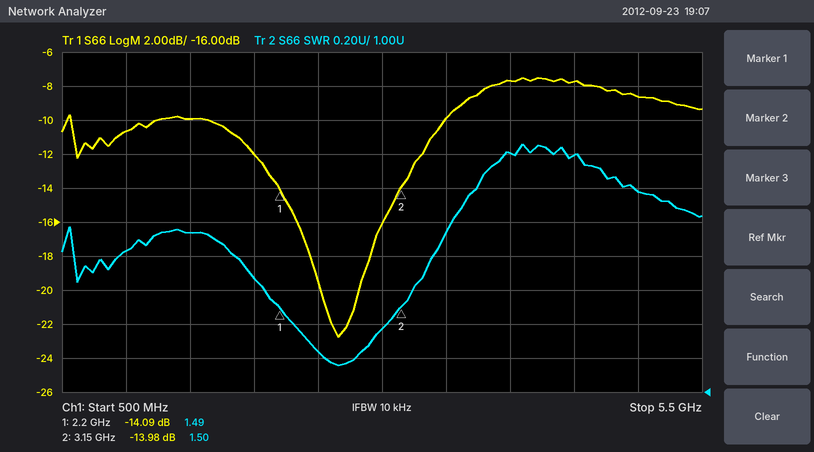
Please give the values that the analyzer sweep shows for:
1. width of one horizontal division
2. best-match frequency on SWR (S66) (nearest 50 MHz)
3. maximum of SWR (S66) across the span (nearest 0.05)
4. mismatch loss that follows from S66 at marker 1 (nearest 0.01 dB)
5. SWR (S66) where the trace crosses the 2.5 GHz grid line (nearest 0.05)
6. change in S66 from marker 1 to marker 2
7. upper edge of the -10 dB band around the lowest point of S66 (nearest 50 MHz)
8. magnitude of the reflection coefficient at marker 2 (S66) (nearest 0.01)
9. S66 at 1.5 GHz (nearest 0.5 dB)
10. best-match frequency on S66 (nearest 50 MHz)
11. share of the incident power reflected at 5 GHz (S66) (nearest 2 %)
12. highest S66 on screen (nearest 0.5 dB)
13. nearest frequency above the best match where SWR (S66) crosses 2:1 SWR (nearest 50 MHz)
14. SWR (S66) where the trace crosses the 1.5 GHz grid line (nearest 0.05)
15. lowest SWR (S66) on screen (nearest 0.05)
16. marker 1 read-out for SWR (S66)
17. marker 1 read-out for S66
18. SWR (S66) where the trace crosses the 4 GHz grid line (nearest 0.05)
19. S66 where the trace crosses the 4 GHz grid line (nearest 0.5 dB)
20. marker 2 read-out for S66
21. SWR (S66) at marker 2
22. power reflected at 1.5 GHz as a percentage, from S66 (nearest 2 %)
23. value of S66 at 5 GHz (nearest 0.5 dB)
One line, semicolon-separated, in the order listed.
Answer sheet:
500 MHz; 2.65 GHz; 2.45; 0.17 dB; 1.25; 0.11 dB; 3.50 GHz; 0.20; -10.0 dB; 2.65 GHz; 14 %; -7.5 dB; 3.55 GHz; 1.95; 1.15; 1.49; -14.09 dB; 2.40; -7.5 dB; -13.98 dB; 1.50; 10 %; -8.5 dB
